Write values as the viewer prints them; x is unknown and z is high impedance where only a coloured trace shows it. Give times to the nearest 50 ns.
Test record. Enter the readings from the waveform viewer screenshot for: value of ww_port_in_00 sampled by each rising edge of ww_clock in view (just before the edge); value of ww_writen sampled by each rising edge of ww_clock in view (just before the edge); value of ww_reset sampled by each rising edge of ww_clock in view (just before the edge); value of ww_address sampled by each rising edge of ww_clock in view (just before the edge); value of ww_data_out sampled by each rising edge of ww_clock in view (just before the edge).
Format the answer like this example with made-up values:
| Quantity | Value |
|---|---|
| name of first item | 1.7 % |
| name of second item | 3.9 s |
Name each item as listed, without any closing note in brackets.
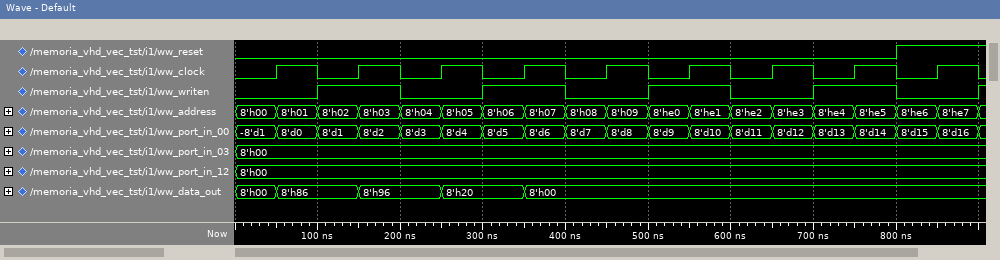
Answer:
| Quantity | Value |
|---|---|
| value of ww_port_in_00 sampled by each rising edge of ww_clock in view | -8'd1, 8'd1, 8'd3, 8'd5, 8'd7, 8'd9, 8'd11, 8'd13, 8'd15 |
| value of ww_writen sampled by each rising edge of ww_clock in view | 0 1 0 1 0 1 0 1 0 |
| value of ww_reset sampled by each rising edge of ww_clock in view | 0 0 0 0 0 0 0 0 1 |
| value of ww_address sampled by each rising edge of ww_clock in view | 8'h00, 8'h02, 8'h04, 8'h06, 8'h08, 8'he0, 8'he2, 8'he4, 8'he6 |
| value of ww_data_out sampled by each rising edge of ww_clock in view | 8'h00, 8'h86, 8'h96, 8'h20, 8'h00, 8'h00, 8'h00, 8'h00, 8'h00 |
